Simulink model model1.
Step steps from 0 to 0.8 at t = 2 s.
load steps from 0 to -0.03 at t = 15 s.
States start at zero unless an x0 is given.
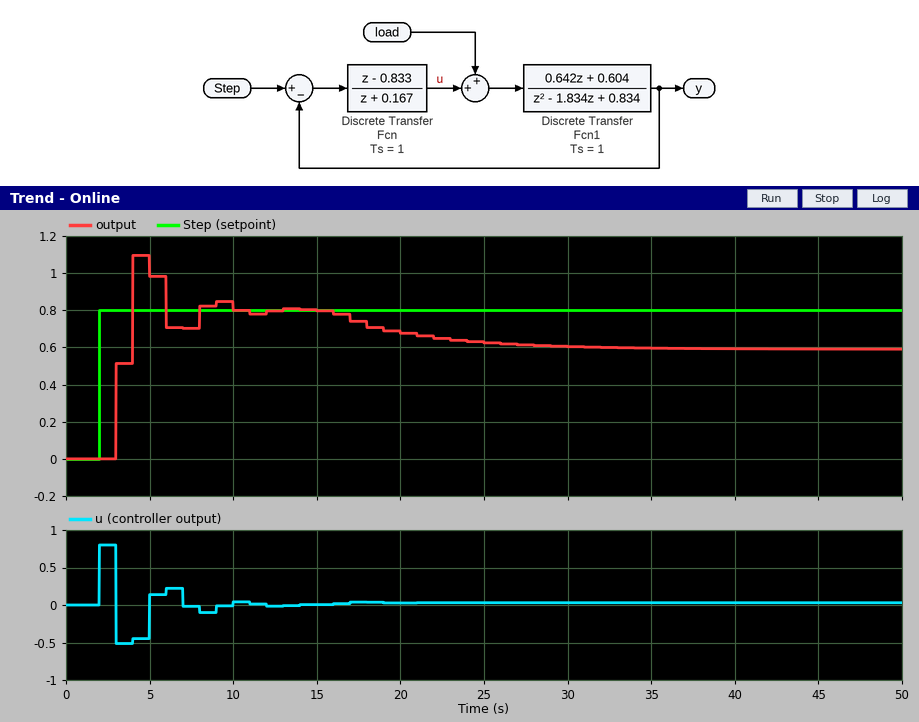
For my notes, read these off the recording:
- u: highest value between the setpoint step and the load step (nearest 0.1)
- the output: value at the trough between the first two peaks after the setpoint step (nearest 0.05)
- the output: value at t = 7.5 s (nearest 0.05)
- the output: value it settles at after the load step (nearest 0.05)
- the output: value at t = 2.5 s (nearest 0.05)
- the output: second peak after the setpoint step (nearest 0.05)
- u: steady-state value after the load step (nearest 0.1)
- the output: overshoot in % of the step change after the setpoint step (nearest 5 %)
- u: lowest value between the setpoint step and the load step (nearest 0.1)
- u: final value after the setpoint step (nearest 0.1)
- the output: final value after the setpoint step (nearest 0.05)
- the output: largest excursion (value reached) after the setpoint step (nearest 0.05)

0.8
0.70
0.70
0.60
0.00
0.85
0.0
35 %
-0.5
0.0
0.80
1.10
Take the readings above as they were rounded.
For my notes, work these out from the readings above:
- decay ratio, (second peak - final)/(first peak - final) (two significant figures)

0.17
